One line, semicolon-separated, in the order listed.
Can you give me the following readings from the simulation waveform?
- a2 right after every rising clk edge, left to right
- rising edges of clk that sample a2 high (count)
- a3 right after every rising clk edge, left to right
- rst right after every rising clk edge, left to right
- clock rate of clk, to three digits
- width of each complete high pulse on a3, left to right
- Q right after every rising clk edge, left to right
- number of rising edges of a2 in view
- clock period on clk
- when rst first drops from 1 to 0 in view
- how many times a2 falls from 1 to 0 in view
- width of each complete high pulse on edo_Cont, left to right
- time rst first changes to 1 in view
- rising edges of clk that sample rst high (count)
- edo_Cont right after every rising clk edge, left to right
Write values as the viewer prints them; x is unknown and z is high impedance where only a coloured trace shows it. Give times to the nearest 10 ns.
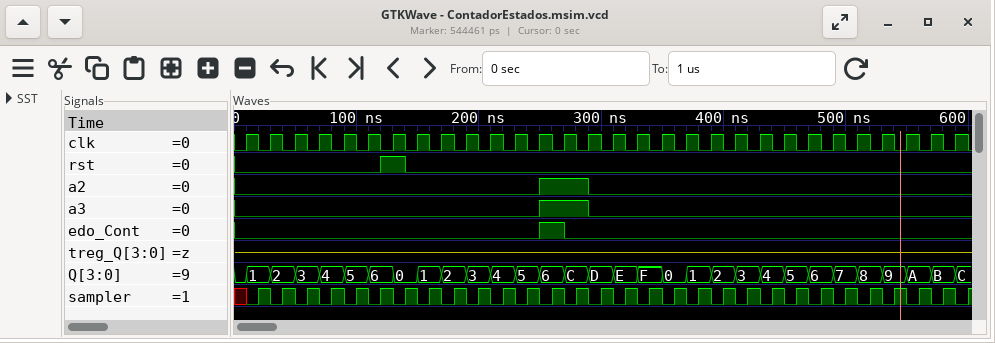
0 0 0 0 0 0 0 0 0 0 0 0 1 1 0 0 0 0 0 0 0 0 0 0 0 0 0 0 0 0; 2; 0 0 0 0 0 0 0 0 0 0 0 0 1 1 0 0 0 0 0 0 0 0 0 0 0 0 0 0 0 0; 0 0 0 0 0 0 1 0 0 0 0 0 0 0 0 0 0 0 0 0 0 0 0 0 0 0 0 0 0 0; 50.0 MHz; 40 ns; 1, 2, 3, 4, 5, 6, 0, 1, 2, 3, 4, 5, 6, C, D, E, F, 0, 1, 2, 3, 4, 5, 6, 7, 8, 9, A, B, C; 1; 20 ns; 140 ns; 1; 20 ns; 120 ns; 1; 0 0 0 0 0 0 0 0 0 0 0 0 1 0 0 0 0 0 0 0 0 0 0 0 0 0 0 0 0 0
